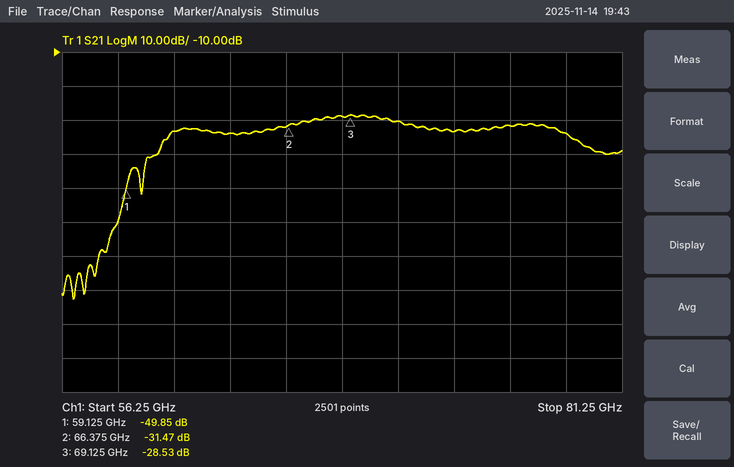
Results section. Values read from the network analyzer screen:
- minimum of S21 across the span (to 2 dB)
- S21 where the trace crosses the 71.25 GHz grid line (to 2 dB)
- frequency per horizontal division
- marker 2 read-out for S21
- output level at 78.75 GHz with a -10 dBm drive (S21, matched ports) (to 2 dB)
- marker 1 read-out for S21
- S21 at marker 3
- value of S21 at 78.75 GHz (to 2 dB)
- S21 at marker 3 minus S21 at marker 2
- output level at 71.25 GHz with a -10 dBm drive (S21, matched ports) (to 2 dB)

-82 dB
-30 dB
2.5 GHz
-31.47 dB
-44 dBm
-49.85 dB
-28.53 dB
-34 dB
2.94 dB
-40 dBm
